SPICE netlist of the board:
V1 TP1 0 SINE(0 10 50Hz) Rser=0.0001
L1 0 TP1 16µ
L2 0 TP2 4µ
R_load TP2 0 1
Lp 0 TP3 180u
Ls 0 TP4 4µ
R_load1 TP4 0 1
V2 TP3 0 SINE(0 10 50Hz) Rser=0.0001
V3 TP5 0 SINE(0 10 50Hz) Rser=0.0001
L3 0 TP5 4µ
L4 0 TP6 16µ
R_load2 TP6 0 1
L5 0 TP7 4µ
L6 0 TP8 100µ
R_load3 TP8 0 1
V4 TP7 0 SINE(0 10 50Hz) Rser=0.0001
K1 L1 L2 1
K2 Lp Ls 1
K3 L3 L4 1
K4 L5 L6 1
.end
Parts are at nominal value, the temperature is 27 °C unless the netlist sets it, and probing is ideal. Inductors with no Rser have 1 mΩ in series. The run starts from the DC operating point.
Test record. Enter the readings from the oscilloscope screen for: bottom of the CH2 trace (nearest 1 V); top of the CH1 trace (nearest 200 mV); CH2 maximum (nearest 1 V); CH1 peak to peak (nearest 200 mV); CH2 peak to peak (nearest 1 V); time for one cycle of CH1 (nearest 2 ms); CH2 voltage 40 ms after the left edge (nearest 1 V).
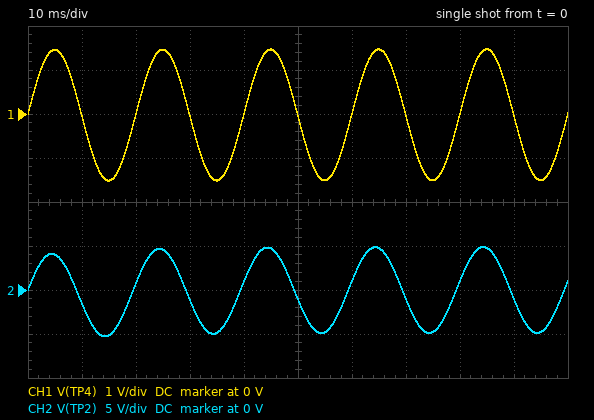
-5 V
1.4 V
5 V
3.0 V
10 V
20 ms
1 V
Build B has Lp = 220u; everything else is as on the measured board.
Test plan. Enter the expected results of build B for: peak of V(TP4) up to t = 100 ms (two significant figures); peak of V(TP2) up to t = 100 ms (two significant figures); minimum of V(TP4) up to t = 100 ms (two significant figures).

1.3 V
4.9 V
-1.4 V
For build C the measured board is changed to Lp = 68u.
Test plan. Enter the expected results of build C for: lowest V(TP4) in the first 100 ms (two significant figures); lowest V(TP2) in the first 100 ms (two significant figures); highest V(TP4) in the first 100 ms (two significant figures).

-2.5 V
-5.3 V
2.4 V
